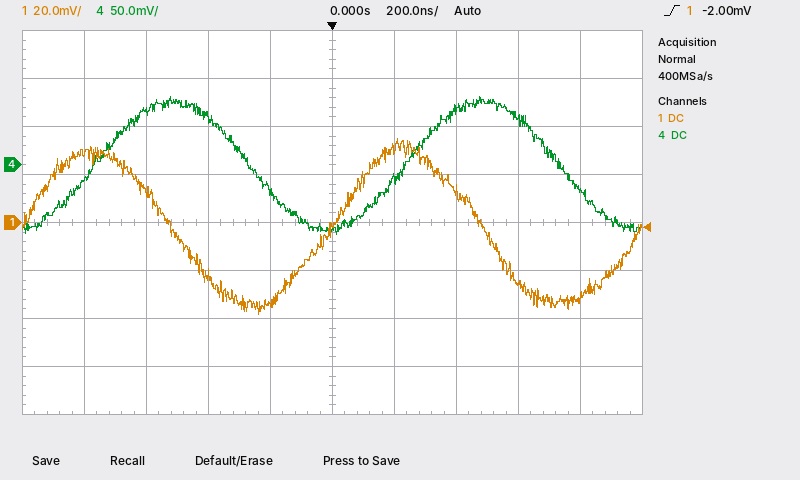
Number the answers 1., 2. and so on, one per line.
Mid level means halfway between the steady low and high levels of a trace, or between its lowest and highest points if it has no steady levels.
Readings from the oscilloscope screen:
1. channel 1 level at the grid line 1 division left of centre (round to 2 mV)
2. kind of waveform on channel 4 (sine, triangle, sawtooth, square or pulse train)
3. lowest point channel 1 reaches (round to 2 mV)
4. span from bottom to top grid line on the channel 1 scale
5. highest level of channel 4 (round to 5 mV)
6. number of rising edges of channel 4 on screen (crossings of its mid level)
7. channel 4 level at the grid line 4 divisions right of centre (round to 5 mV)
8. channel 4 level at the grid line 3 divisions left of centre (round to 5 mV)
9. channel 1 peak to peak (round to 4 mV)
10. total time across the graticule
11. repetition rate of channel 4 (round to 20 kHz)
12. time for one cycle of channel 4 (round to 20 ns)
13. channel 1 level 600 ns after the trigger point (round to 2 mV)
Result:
1. -34 mV
2. sine
3. -38 mV
4. 160 mV
5. 70 mV
6. 2
7. -25 mV
8. 55 mV
9. 72 mV
10. 2 µs
11. 1.00 MHz
12. 1.00 µs
13. -26 mV
